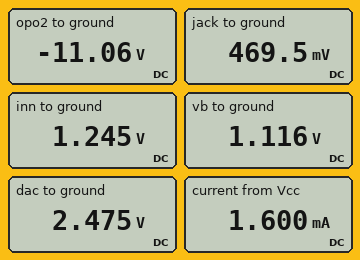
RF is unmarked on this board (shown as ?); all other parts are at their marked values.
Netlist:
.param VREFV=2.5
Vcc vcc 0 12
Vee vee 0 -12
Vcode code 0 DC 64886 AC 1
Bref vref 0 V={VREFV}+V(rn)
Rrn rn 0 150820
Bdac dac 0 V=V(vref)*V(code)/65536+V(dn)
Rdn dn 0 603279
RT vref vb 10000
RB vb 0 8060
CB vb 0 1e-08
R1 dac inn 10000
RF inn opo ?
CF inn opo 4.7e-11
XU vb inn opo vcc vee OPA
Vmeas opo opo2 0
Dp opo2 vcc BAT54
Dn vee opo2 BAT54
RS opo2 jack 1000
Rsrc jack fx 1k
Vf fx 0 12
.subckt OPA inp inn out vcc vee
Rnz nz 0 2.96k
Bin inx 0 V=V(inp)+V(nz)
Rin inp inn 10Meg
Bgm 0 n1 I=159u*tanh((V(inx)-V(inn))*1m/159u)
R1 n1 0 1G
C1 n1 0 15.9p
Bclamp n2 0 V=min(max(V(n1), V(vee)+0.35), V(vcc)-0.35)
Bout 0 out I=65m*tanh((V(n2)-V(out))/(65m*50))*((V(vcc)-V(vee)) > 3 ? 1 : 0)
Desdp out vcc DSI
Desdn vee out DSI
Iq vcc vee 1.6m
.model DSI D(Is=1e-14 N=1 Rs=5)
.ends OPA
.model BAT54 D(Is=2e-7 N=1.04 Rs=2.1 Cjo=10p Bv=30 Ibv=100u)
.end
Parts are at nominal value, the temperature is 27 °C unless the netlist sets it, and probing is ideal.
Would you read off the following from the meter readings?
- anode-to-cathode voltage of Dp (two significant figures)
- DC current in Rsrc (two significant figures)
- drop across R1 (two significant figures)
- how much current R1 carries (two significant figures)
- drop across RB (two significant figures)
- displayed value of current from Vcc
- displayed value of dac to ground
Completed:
-23 V
12 mA
1.2 V
120 µA
1.1 V
1.600 mA
2.475 V
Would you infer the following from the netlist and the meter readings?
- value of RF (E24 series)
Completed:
100 kΩ
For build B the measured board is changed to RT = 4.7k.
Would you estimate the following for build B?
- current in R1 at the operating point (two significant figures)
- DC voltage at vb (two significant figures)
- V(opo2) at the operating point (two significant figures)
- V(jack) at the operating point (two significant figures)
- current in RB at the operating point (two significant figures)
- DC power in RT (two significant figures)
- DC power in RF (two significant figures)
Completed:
90 µA
1.6 V
-7.4 V
2.3 V
200 µA
180 µW
800 µW
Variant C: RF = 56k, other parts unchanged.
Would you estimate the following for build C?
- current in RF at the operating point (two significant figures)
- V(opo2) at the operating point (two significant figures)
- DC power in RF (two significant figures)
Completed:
140 µA
-6.5 V
1.0 mW
